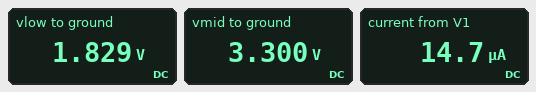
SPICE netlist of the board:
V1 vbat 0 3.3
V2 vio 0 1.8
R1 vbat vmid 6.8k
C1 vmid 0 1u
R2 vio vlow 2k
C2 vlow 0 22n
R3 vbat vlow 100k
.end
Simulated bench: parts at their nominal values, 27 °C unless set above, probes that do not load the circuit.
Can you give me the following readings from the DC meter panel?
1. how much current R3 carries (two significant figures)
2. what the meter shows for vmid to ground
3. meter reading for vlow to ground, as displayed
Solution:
15 µA
3.300 V
1.829 V
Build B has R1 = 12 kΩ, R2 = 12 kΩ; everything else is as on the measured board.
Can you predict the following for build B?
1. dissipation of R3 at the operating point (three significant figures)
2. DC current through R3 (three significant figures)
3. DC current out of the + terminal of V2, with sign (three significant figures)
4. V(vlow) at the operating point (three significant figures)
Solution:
17.9 µW
13.4 µA
-13.4 µA
1.96 V
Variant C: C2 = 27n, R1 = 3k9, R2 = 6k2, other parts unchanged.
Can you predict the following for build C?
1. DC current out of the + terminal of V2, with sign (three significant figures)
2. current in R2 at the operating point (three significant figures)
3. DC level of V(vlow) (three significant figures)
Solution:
-14.1 µA
14.1 µA
1.89 V
